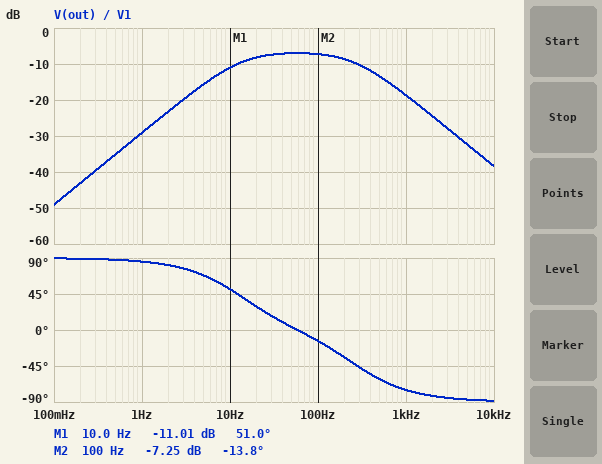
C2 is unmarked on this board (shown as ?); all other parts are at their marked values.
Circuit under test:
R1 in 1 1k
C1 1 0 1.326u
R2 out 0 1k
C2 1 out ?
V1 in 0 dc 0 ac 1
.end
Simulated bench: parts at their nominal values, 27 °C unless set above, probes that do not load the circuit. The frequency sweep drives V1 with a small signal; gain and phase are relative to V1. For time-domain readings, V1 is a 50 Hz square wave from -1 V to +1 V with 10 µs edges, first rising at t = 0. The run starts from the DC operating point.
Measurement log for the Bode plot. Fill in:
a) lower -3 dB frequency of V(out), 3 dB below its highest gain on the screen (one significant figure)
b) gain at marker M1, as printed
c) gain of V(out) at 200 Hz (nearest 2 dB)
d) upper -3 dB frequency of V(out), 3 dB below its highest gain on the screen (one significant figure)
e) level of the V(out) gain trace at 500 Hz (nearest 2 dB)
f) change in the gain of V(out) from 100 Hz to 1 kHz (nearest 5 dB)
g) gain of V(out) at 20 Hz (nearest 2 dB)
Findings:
10 Hz
-11.01 dB
-8 dB
300 Hz
-14 dB
-10 dB
-8 dB
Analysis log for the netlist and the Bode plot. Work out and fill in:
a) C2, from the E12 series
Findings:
5.6 µF
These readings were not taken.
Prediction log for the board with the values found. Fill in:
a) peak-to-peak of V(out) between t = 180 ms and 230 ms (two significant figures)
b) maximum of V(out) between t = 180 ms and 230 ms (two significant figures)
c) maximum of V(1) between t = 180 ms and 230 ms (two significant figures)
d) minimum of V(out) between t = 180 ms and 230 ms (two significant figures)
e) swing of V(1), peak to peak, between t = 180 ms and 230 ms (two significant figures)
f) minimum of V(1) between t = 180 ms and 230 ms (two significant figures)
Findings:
1.1 V
550 mV
660 mV
-550 mV
1.3 V
-660 mV
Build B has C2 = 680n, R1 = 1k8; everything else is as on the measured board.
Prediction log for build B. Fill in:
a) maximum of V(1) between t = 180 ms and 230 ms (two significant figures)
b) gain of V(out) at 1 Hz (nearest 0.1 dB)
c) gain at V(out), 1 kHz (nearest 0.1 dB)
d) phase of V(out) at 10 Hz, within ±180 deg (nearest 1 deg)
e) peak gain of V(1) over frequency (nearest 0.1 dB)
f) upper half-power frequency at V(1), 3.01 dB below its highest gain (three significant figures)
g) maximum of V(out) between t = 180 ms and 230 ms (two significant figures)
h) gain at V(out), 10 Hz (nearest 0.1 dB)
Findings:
870 mV
-47.4 dB
-24.1 dB
75 deg
0 dB
41.9 Hz
250 mV
-27.6 dB
